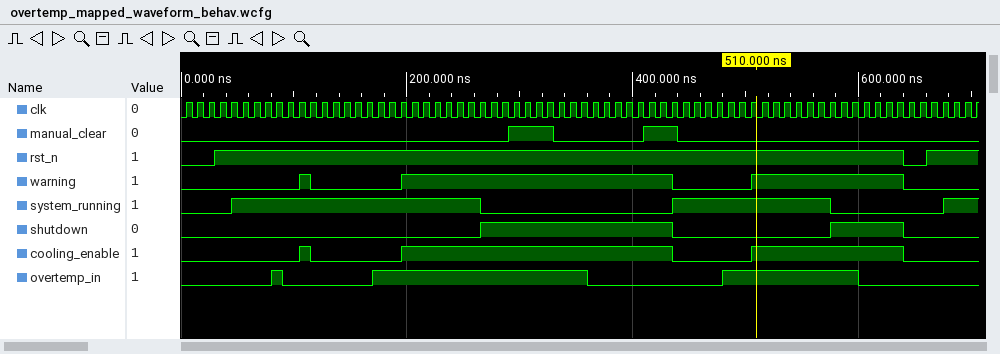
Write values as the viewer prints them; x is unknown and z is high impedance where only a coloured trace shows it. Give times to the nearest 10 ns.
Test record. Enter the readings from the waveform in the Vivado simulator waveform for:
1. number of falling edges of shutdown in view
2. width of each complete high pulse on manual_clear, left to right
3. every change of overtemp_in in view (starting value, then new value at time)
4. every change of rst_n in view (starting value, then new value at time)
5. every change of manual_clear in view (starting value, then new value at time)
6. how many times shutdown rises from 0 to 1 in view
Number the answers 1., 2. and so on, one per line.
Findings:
1. 2
2. 40 ns, 30 ns
3. 0, 1 at 80 ns, 0 at 90 ns, 1 at 170 ns, 0 at 360 ns, 1 at 480 ns, 0 at 600 ns
4. 0, 1 at 30 ns, 0 at 640 ns, 1 at 660 ns
5. 0, 1 at 290 ns, 0 at 330 ns, 1 at 410 ns, 0 at 440 ns
6. 2
